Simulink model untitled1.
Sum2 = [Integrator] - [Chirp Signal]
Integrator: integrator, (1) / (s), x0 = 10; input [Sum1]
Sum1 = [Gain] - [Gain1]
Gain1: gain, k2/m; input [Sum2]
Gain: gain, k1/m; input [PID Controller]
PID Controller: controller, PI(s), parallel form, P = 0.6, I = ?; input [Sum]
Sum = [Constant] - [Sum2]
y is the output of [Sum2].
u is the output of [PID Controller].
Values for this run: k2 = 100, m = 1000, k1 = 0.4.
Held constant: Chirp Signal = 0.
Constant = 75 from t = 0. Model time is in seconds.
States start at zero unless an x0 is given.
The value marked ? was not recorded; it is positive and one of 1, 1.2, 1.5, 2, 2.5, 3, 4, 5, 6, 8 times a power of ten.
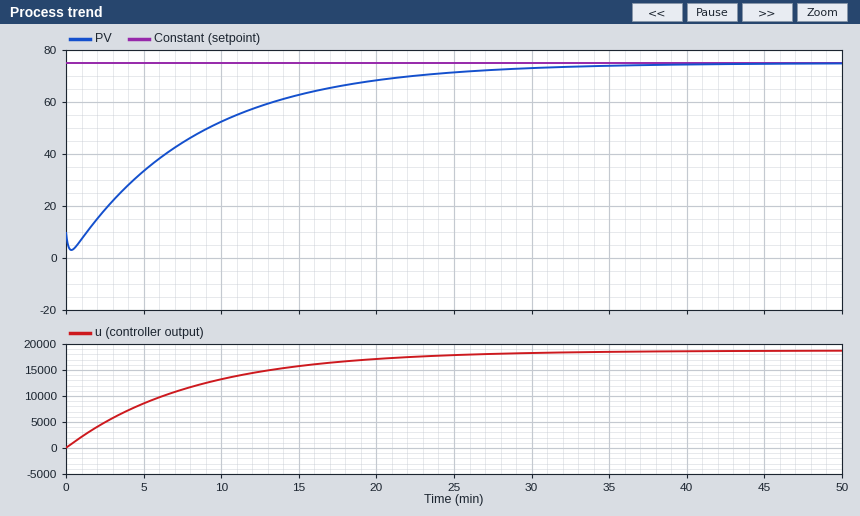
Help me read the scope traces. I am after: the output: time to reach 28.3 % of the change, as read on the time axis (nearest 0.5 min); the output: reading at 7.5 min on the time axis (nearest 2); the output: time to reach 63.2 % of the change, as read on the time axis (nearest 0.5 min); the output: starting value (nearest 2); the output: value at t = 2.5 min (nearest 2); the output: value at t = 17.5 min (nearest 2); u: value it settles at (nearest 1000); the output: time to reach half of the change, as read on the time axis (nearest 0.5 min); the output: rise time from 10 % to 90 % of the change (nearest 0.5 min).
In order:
4.0 min
44
9.5 min
10
18
66
19000
7.0 min
18.0 min
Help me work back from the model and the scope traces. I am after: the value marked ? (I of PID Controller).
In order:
0.5
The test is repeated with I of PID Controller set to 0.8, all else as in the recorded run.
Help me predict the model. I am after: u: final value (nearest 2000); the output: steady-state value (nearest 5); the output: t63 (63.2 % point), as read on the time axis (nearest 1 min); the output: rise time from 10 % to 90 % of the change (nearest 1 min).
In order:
18000
75
6 min
11 min
